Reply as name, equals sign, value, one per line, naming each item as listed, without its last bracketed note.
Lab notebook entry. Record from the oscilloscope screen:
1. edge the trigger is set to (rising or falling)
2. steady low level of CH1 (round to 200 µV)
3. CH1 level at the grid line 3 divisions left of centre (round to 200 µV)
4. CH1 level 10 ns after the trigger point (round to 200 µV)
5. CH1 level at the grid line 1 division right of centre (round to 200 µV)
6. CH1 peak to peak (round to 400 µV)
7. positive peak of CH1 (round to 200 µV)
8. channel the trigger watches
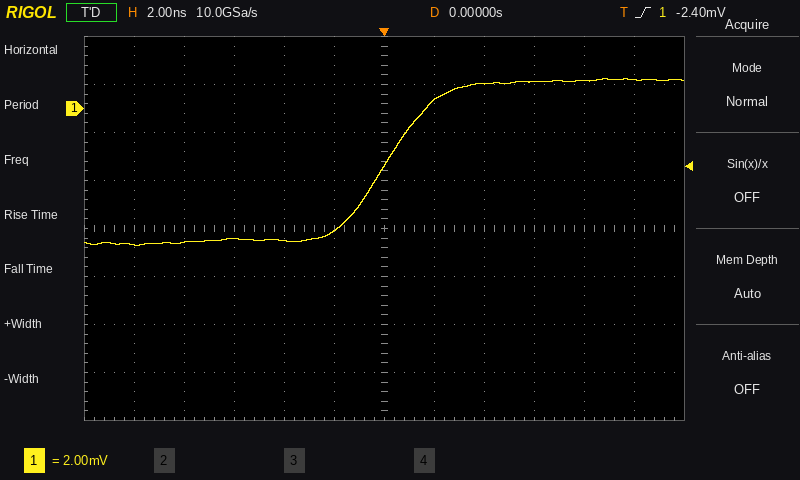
edge the trigger is set to = rising
steady low level of CH1 = -5.6 mV
CH1 level at the grid line 3 divisions left of centre = -5.4 mV
CH1 level 10 ns after the trigger point = 1.2 mV
CH1 level at the grid line 1 division right of centre = 400 µV
CH1 peak to peak = 6.8 mV
positive peak of CH1 = 1.2 mV
channel the trigger watches = CH1
